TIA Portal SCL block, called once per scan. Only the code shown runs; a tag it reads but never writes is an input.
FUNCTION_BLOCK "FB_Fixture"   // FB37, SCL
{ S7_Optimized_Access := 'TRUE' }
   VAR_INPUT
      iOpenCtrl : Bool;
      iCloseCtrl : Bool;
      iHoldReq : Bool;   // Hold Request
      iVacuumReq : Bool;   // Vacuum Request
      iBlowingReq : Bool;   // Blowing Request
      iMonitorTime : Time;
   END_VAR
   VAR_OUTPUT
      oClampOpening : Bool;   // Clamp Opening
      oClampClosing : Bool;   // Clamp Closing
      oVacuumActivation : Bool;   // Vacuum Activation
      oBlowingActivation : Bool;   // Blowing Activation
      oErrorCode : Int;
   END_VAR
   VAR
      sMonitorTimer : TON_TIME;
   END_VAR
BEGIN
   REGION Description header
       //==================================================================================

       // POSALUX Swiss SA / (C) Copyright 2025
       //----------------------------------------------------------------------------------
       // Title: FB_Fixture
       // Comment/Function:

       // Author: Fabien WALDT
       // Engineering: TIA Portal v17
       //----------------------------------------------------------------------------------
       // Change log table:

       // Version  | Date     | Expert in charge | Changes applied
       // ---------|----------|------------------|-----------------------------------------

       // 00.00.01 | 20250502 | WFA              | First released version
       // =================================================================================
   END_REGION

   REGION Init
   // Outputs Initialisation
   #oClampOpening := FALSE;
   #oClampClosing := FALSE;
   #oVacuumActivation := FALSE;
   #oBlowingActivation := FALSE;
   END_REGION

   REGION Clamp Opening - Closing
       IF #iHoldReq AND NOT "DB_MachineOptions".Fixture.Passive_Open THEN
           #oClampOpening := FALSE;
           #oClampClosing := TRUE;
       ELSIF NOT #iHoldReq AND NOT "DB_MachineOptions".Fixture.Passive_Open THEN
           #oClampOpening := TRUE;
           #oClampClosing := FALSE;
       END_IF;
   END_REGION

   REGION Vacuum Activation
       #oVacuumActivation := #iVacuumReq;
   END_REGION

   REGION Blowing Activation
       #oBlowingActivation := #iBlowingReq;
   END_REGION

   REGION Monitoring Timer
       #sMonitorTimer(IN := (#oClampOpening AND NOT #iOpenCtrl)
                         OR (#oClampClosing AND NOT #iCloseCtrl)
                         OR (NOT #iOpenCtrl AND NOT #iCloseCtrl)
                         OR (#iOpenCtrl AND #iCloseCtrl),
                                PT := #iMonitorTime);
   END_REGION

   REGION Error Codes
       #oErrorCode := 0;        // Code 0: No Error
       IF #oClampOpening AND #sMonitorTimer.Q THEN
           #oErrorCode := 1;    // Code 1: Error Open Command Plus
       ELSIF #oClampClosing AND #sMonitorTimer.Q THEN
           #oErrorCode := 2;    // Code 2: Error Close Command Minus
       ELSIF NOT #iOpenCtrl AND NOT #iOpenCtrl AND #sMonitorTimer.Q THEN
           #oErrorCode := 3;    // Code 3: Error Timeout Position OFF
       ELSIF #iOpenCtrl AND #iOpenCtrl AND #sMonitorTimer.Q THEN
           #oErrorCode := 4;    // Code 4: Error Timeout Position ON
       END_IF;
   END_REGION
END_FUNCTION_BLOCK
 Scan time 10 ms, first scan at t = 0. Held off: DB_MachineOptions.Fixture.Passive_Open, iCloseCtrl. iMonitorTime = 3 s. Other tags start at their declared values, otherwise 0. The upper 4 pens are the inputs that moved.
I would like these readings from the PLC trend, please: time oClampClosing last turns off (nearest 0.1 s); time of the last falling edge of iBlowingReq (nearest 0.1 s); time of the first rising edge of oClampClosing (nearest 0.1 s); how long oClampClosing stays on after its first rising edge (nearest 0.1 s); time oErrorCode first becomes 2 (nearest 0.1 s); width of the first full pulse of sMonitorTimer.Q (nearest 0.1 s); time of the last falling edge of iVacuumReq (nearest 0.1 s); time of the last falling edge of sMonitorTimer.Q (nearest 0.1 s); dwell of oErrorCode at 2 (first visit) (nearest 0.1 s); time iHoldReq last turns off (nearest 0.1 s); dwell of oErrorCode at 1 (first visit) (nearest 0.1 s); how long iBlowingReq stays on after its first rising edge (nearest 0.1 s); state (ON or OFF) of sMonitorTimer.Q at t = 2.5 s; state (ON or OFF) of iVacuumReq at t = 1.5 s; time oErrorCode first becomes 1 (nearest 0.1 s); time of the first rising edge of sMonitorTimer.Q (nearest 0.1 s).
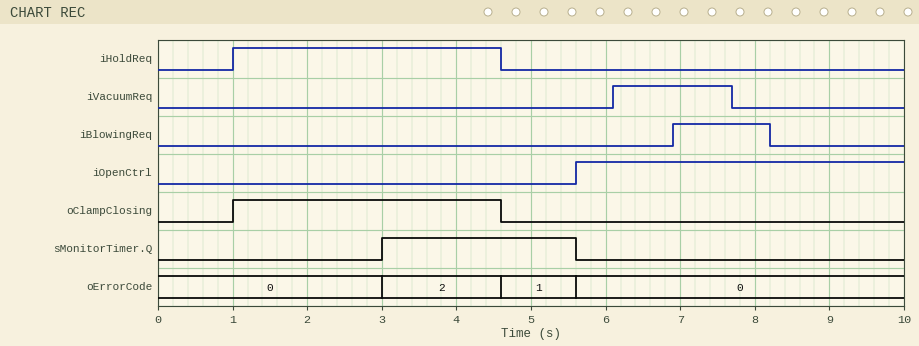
4.6 s
8.2 s
1.0 s
3.6 s
3.0 s
2.6 s
7.7 s
5.6 s
1.6 s
4.6 s
1.0 s
1.3 s
OFF
OFF
4.6 s
3.0 s
